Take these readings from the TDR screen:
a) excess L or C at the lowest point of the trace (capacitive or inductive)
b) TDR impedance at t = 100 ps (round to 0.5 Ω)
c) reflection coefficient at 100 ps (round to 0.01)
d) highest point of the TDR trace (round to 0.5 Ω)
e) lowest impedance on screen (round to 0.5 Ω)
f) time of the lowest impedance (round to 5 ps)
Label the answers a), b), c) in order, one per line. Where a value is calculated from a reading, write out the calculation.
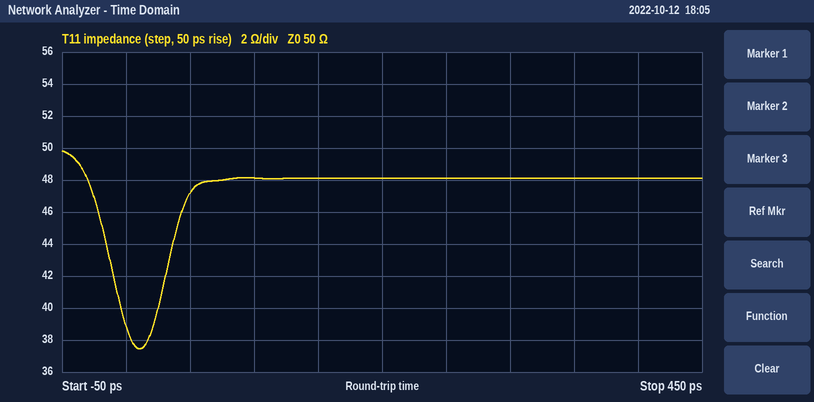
a) capacitive
b) 48.0 Ω
c) (48 − 50)/(48 + 50) ≈ -0.02
d) 50.0 Ω
e) 37.5 Ω
f) 10 ps
